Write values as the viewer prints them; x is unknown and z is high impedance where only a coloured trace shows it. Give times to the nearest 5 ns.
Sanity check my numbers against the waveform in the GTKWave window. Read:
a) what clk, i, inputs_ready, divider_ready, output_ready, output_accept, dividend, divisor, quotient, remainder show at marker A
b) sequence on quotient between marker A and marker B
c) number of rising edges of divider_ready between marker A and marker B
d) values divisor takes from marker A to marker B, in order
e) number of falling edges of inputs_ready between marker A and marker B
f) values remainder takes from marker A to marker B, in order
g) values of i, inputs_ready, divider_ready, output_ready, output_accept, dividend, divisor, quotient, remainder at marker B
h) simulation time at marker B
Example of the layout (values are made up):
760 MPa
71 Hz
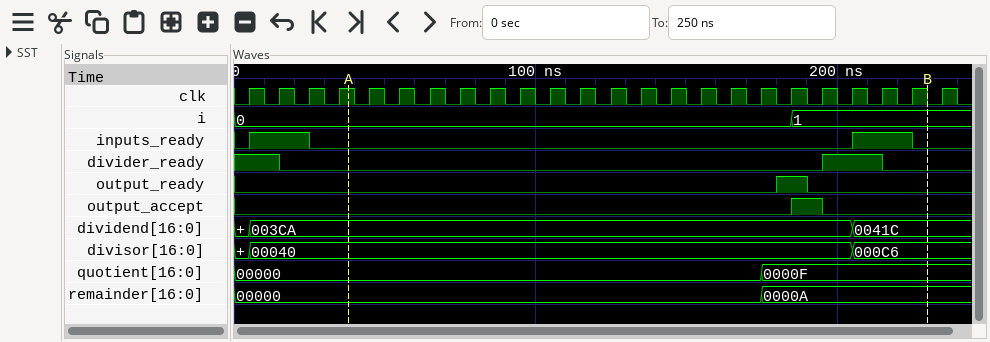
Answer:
clk=1, i=0, inputs_ready=0, divider_ready=0, output_ready=0, output_accept=0, dividend=003CA, divisor=00040, quotient=00000, remainder=00000
00000, 0000F
1
00040, 000C6
1
00000, 0000A
i=1, inputs_ready=0, divider_ready=0, output_ready=0, output_accept=0, dividend=0041C, divisor=000C6, quotient=0000F, remainder=0000A
230 ns
